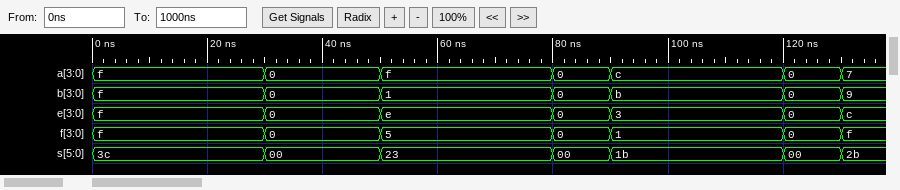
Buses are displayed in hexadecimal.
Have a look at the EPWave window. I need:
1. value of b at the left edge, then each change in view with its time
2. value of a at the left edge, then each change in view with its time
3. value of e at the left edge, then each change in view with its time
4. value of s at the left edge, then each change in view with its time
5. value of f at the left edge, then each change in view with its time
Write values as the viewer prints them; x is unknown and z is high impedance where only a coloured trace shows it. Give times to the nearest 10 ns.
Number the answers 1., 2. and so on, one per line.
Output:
1. f, 0 at 30 ns, 1 at 50 ns, 0 at 80 ns, b at 90 ns, 0 at 120 ns, 9 at 130 ns
2. f, 0 at 30 ns, f at 50 ns, 0 at 80 ns, c at 90 ns, 0 at 120 ns, 7 at 130 ns
3. f, 0 at 30 ns, e at 50 ns, 0 at 80 ns, 3 at 90 ns, 0 at 120 ns, c at 130 ns
4. 3c, 00 at 30 ns, 23 at 50 ns, 00 at 80 ns, 1b at 90 ns, 00 at 120 ns, 2b at 130 ns
5. f, 0 at 30 ns, 5 at 50 ns, 0 at 80 ns, 1 at 90 ns, 0 at 120 ns, f at 130 ns
